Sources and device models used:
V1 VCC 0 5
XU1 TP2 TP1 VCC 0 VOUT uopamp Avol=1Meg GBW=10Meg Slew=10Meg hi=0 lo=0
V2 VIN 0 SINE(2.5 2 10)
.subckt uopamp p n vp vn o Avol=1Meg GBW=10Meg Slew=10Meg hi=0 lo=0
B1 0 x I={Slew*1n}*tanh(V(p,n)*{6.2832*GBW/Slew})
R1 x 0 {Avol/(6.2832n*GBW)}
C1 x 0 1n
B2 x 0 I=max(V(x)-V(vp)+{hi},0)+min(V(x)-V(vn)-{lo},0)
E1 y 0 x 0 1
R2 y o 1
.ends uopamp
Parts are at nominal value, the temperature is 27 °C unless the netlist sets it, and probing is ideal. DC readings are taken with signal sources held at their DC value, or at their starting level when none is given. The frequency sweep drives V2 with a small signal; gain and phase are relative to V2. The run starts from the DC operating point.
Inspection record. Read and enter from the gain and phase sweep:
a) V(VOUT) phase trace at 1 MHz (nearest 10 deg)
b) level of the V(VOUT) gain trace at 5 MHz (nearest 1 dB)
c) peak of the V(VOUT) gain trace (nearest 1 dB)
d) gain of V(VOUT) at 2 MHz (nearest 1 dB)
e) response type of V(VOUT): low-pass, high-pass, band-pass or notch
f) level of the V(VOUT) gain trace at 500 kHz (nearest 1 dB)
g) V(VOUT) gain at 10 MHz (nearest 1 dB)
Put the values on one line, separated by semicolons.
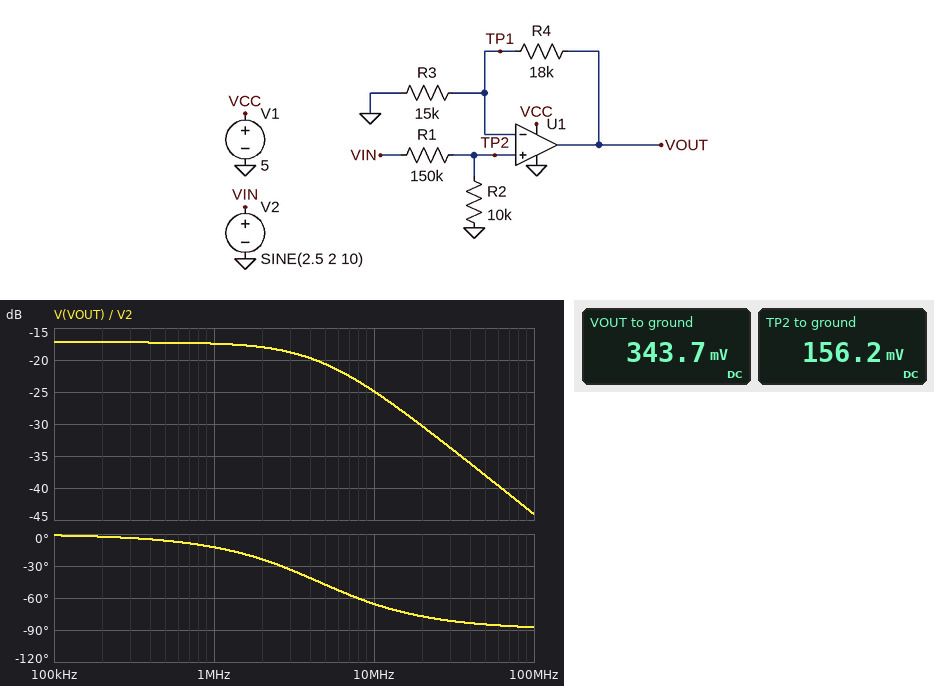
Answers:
-10 deg; -21 dB; -17 dB; -18 dB; low-pass; -17 dB; -25 dB
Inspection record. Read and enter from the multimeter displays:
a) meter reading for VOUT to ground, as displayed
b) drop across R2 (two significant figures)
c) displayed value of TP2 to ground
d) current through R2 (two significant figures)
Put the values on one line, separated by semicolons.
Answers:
343.7 mV; 160 mV; 156.2 mV; 16 µA
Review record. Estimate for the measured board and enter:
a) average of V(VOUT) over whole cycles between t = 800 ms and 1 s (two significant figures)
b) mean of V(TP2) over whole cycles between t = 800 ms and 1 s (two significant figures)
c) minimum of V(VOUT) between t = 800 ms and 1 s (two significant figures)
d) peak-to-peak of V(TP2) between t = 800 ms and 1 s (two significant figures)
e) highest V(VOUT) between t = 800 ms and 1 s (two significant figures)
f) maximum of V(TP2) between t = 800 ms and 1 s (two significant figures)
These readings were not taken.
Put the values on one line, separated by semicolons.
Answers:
340 mV; 160 mV; 69 mV; 250 mV; 620 mV; 280 mV
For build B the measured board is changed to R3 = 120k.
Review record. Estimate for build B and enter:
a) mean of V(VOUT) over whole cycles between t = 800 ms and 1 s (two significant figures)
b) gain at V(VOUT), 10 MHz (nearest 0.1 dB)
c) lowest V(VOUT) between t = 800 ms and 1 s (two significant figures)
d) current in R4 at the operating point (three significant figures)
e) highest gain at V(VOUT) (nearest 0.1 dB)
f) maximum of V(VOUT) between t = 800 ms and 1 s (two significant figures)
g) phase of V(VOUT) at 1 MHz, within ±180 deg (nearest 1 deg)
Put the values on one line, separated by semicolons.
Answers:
180 mV; -26.5 dB; 36 mV; 1.30 µA; -22.9 dB; 320 mV; -7 deg
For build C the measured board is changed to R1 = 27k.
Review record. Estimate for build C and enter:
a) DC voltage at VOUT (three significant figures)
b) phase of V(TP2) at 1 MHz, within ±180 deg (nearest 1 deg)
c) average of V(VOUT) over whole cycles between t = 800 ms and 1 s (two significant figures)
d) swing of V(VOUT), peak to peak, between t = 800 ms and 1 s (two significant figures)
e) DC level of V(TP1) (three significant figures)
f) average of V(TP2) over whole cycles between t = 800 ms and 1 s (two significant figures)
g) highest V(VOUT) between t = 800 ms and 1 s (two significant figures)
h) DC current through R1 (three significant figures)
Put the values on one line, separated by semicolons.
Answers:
1.49 V; 0 deg; 1.5 V; 2.4 V; 676 mV; 680 mV; 2.7 V; 67.6 µA
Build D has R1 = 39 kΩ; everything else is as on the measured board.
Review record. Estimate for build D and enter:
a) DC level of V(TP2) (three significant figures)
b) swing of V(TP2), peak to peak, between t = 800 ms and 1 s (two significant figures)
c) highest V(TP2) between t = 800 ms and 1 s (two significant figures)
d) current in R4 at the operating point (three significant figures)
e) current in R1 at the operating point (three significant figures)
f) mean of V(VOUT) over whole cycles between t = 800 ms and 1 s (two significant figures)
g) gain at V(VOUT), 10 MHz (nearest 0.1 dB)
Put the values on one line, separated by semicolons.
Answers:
510 mV; 820 mV; 920 mV; 34.0 µA; 51.0 µA; 1.1 V; -14.6 dB
